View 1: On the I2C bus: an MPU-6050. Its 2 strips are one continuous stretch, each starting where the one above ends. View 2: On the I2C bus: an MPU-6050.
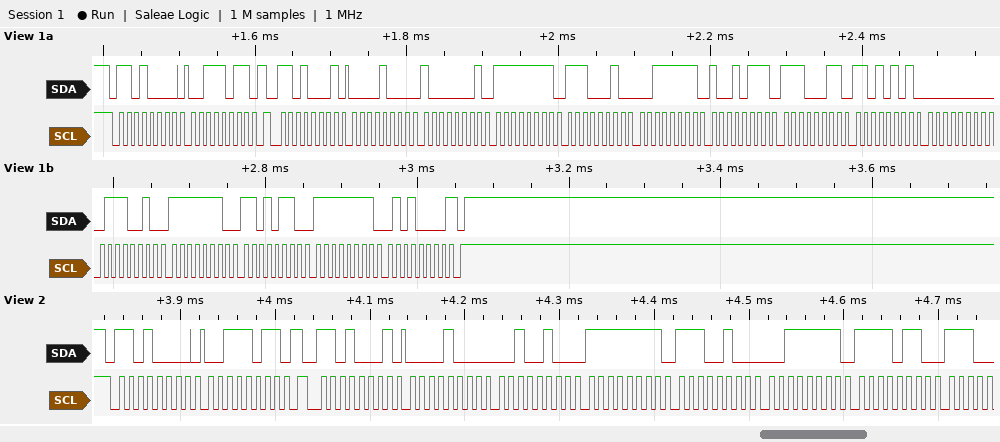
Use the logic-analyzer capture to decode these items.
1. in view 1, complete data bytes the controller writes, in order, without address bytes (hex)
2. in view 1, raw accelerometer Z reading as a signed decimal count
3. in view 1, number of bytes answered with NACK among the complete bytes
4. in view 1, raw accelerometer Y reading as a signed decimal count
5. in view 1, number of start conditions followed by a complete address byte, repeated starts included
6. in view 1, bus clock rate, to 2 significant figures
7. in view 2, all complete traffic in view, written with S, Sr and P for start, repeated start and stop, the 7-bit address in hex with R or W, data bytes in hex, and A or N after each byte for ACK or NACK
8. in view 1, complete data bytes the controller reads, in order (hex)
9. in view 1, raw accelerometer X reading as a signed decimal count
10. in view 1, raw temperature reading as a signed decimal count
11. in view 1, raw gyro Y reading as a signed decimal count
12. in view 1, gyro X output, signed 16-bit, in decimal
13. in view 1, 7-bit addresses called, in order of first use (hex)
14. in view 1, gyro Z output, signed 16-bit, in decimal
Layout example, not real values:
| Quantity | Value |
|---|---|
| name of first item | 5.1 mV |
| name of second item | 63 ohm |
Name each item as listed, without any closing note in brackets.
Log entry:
| Quantity | Value |
|---|---|
| in view 1, complete data bytes the controller writes, in order, without address bytes | 3B |
| in view 1, raw accelerometer Z reading as a signed decimal count | 16279 |
| in view 1, number of bytes answered with NACK among the complete bytes | 1 |
| in view 1, raw accelerometer Y reading as a signed decimal count | -30 |
| in view 1, number of start conditions followed by a complete address byte, repeated starts included | 2 |
| in view 1, bus clock rate, to 2 significant figures | 100 kHz |
| in view 2, all complete traffic in view, written with S, Sr and P for start, repeated start and stop, the 7-bit address in hex with R or W, data bytes in hex, and A or N after each byte for ACK or NACK | S 68W A 3B A Sr 68R A 08 A 24 A FF A E4 A 3F A F6 A |
| in view 1, complete data bytes the controller reads, in order | 08 81 FF E2 3F 97 E3 D5 00 72 FE D6 FF 50 |
| in view 1, raw accelerometer X reading as a signed decimal count | 2177 |
| in view 1, raw temperature reading as a signed decimal count | -7211 |
| in view 1, raw gyro Y reading as a signed decimal count | -298 |
| in view 1, gyro X output, signed 16-bit, in decimal | 114 |
| in view 1, 7-bit addresses called, in order of first use | 0x68 |
| in view 1, gyro Z output, signed 16-bit, in decimal | -176 |
